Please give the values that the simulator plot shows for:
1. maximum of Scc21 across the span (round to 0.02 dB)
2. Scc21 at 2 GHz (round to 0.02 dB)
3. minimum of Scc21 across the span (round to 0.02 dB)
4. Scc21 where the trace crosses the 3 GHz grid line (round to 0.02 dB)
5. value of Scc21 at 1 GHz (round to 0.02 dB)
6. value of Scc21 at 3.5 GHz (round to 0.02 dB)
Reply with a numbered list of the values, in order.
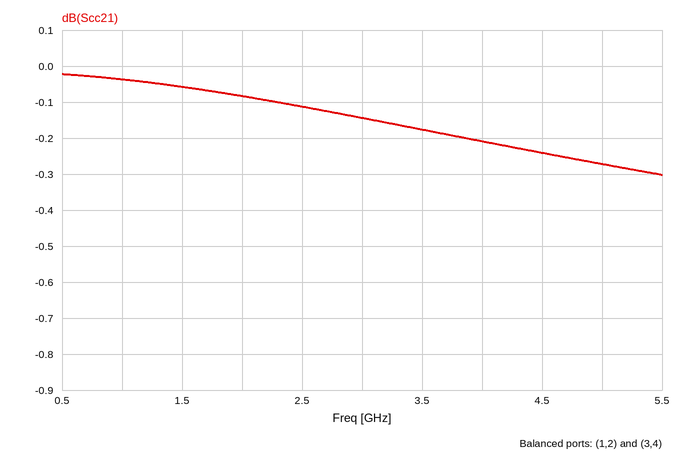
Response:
1. -0.02 dB
2. -0.08 dB
3. -0.30 dB
4. -0.14 dB
5. -0.04 dB
6. -0.18 dB
